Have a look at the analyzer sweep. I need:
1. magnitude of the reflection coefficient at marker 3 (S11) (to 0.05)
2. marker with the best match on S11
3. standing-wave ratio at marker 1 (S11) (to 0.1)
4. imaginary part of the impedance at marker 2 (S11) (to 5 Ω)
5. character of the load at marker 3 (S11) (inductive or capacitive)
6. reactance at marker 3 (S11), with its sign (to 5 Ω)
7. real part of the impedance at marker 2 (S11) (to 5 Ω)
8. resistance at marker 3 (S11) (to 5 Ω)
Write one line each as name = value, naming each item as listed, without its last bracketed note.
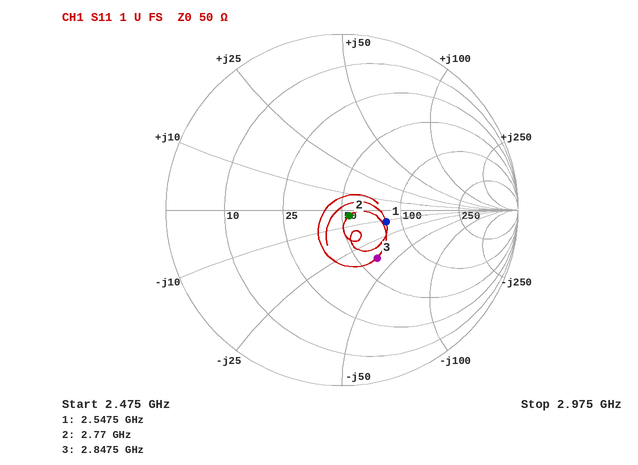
magnitude of the reflection coefficient at marker 3 (S11) = 0.35
marker with the best match on S11 = marker 2
standing-wave ratio at marker 1 (S11) = 1.7
imaginary part of the impedance at marker 2 (S11) = -5 Ω
character of the load at marker 3 (S11) = capacitive
reactance at marker 3 (S11), with its sign = -40 Ω
real part of the impedance at marker 2 (S11) = 55 Ω
resistance at marker 3 (S11) = 60 Ω
